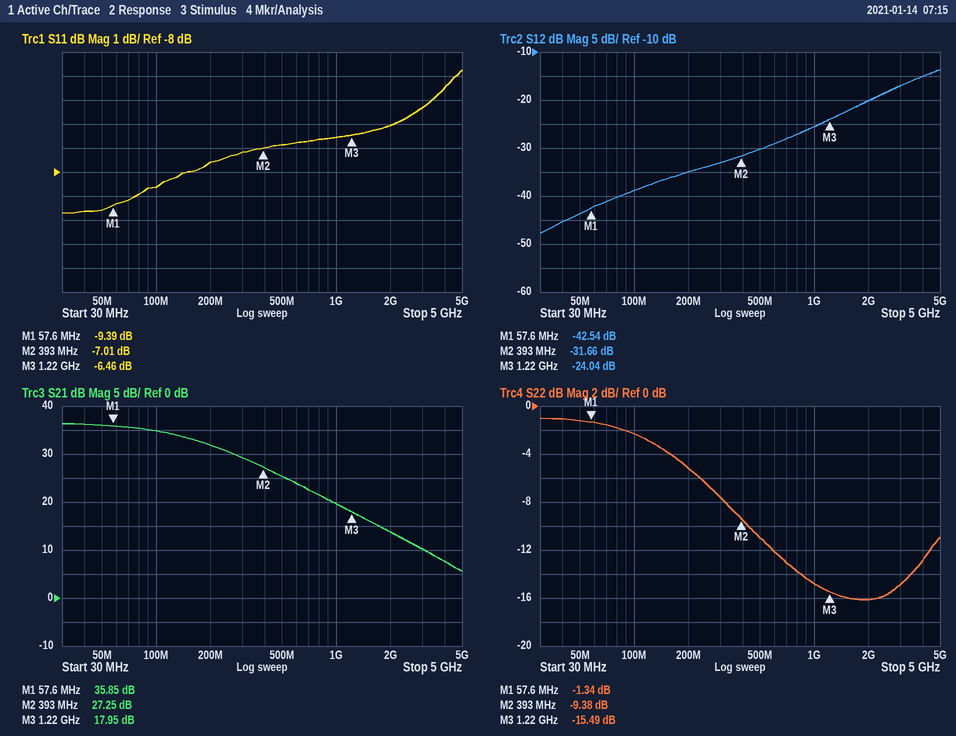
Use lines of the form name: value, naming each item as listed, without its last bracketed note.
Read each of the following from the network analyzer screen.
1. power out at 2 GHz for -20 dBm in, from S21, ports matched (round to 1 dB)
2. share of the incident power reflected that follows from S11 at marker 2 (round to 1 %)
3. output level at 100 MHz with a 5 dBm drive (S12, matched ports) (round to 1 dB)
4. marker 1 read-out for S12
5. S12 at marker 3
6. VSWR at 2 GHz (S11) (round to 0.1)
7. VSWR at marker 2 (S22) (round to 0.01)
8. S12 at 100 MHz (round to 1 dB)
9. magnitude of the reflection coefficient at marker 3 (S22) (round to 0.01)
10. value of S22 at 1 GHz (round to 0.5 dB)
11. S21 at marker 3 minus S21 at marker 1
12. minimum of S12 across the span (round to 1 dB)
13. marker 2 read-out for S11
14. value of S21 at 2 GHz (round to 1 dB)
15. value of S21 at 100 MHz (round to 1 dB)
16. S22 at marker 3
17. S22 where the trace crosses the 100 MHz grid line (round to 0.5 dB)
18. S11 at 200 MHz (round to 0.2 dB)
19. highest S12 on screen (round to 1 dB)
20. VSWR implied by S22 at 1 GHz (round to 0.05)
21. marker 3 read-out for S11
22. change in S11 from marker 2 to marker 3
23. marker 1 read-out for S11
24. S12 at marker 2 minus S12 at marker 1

power out at 2 GHz for -20 dBm in, from S21, ports matched: -6 dBm
share of the incident power reflected that follows from S11 at marker 2: 20 %
output level at 100 MHz with a 5 dBm drive (S12, matched ports): -34 dBm
marker 1 read-out for S12: -42.54 dB
S12 at marker 3: -24.04 dB
VSWR at 2 GHz (S11): 3.0
VSWR at marker 2 (S22): 2.03
S12 at 100 MHz: -39 dB
magnitude of the reflection coefficient at marker 3 (S22): 0.17
value of S22 at 1 GHz: -15.0 dB
S21 at marker 3 minus S21 at marker 1: -17.90 dB
minimum of S12 across the span: -48 dB
marker 2 read-out for S11: -7.01 dB
value of S21 at 2 GHz: 14 dB
value of S21 at 100 MHz: 35 dB
S22 at marker 3: -15.49 dB
S22 where the trace crosses the 100 MHz grid line: -2.5 dB
S11 at 200 MHz: -7.6 dB
highest S12 on screen: -14 dB
VSWR implied by S22 at 1 GHz: 1.45
marker 3 read-out for S11: -6.46 dB
change in S11 from marker 2 to marker 3: 0.55 dB
marker 1 read-out for S11: -9.39 dB
S12 at marker 2 minus S12 at marker 1: 10.88 dB
